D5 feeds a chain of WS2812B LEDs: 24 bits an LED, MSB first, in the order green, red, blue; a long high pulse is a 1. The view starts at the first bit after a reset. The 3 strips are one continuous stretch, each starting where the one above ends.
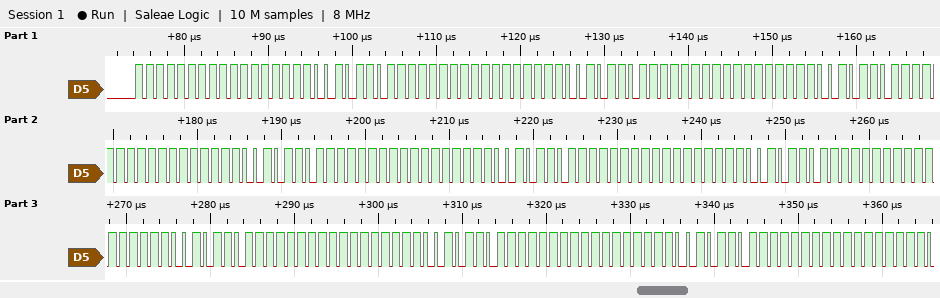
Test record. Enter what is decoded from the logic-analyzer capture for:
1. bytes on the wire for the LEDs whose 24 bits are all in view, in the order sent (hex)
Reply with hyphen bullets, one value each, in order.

- FF FF 96 FF FF 96 FF FF 96 FF FF 96 FF FF 96 FF FF 96 FF FF 96 FF FF 96 FF FF 96
